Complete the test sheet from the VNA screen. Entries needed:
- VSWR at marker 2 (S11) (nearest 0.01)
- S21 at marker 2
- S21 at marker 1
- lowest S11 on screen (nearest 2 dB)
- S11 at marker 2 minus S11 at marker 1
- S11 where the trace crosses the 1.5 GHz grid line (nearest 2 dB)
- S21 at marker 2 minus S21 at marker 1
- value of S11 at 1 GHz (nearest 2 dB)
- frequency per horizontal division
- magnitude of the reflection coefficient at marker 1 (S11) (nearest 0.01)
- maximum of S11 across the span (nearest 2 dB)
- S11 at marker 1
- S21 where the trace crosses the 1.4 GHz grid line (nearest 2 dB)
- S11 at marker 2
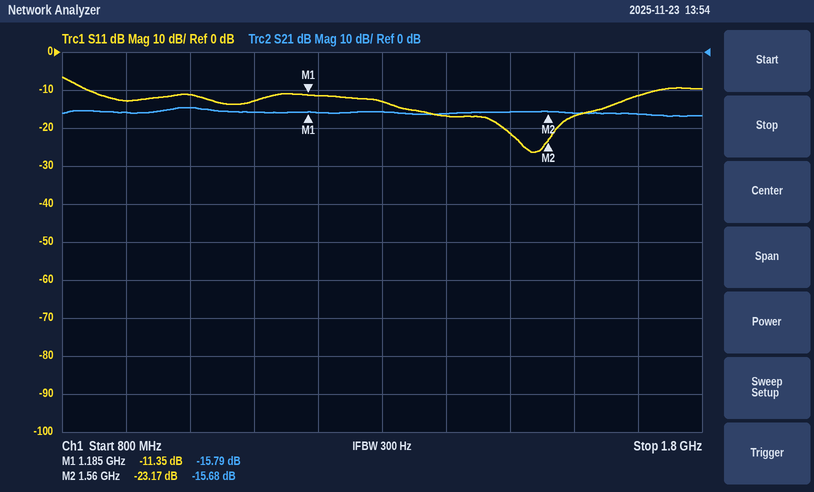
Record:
1.15
-15.68 dB
-15.79 dB
-26 dB
-11.82 dB
-22 dB
0.11 dB
-12 dB
100 MHz
0.27
-6 dB
-11.35 dB
-16 dB
-23.17 dB
